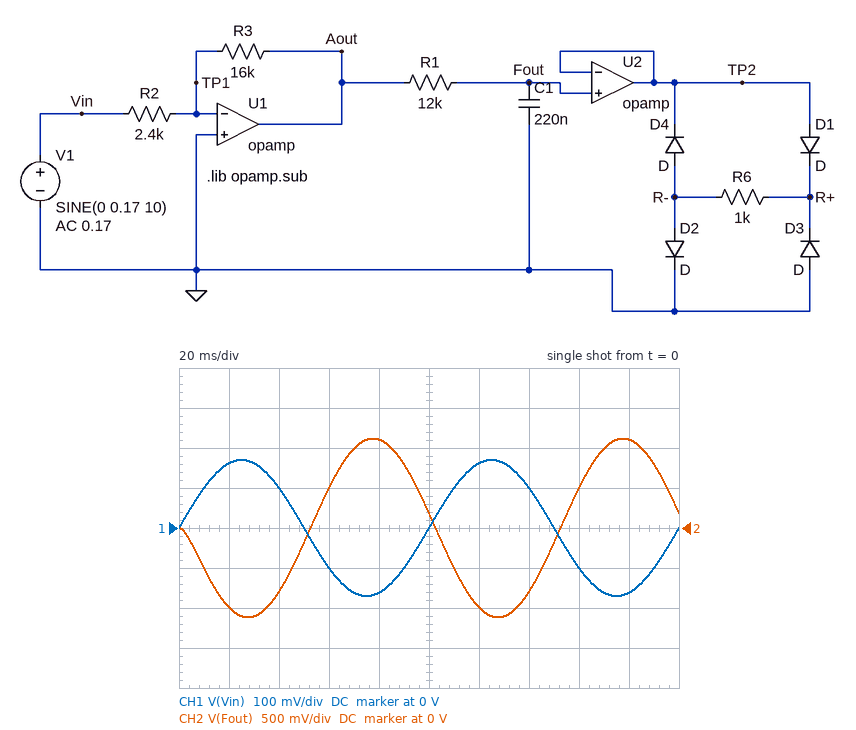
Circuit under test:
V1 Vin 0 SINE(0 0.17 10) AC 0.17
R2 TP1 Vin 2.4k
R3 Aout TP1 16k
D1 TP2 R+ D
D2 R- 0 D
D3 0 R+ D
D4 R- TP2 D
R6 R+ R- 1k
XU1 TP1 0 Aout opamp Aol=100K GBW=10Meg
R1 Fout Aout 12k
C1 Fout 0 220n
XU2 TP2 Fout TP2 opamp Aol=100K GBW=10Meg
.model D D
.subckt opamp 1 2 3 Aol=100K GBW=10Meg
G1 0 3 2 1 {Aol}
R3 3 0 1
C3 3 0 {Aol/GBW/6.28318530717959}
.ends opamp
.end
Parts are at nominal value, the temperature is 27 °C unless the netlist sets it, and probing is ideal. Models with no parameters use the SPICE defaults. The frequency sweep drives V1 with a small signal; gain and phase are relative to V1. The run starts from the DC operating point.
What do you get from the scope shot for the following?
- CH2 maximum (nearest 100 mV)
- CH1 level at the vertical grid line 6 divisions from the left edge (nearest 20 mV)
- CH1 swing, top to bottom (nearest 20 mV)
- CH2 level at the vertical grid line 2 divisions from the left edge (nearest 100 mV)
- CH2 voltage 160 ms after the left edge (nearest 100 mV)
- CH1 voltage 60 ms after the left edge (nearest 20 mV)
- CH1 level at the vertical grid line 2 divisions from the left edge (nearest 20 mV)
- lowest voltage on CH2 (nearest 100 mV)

1.1 V
160 mV
340 mV
-800 mV
500 mV
-100 mV
100 mV
-1.1 V
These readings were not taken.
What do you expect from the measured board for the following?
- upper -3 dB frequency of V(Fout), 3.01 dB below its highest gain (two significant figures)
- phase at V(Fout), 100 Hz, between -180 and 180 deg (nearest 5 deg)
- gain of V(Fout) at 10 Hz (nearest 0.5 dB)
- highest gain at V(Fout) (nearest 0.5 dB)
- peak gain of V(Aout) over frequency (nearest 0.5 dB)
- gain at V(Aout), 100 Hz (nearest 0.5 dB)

60 Hz
120 deg
16.5 dB
16.5 dB
16.5 dB
16.5 dB
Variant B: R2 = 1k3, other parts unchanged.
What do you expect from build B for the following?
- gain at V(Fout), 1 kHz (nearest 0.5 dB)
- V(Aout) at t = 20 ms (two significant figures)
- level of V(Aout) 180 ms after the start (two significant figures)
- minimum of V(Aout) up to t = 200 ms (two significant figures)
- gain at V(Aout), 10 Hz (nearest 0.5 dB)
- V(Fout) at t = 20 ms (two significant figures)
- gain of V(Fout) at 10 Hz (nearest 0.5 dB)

-2.5 dB
-2.0 V
2.0 V
-2.1 V
22.0 dB
-1.8 V
21.5 dB
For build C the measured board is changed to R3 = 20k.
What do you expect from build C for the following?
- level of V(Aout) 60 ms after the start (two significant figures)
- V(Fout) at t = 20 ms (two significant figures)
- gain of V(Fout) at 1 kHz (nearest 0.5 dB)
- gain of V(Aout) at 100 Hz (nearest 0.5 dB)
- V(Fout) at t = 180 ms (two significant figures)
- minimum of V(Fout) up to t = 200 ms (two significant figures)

830 mV
-1.2 V
-6.0 dB
18.5 dB
1.4 V
-1.4 V
